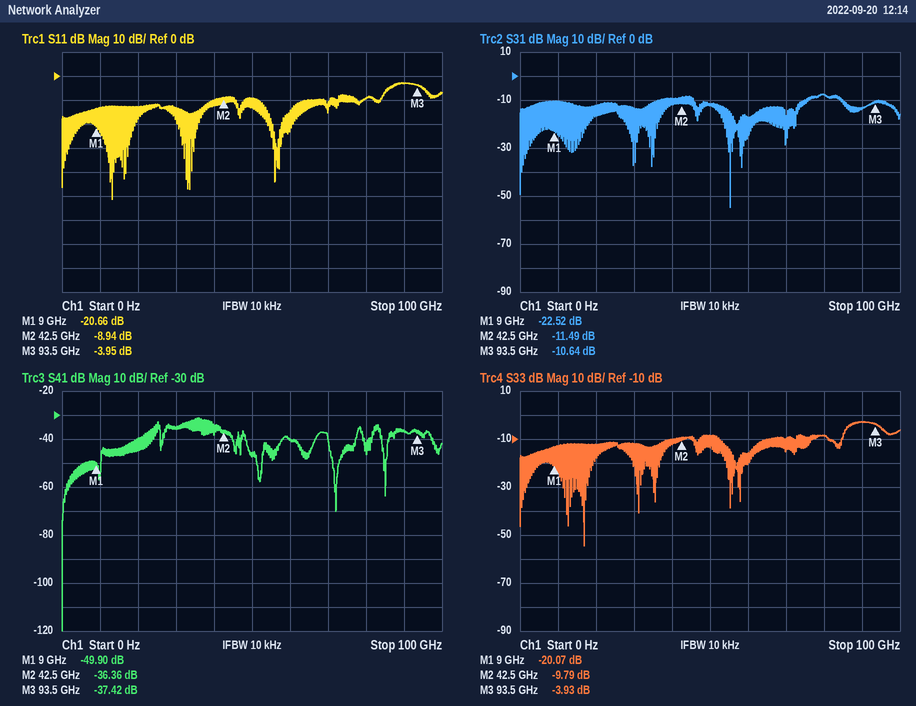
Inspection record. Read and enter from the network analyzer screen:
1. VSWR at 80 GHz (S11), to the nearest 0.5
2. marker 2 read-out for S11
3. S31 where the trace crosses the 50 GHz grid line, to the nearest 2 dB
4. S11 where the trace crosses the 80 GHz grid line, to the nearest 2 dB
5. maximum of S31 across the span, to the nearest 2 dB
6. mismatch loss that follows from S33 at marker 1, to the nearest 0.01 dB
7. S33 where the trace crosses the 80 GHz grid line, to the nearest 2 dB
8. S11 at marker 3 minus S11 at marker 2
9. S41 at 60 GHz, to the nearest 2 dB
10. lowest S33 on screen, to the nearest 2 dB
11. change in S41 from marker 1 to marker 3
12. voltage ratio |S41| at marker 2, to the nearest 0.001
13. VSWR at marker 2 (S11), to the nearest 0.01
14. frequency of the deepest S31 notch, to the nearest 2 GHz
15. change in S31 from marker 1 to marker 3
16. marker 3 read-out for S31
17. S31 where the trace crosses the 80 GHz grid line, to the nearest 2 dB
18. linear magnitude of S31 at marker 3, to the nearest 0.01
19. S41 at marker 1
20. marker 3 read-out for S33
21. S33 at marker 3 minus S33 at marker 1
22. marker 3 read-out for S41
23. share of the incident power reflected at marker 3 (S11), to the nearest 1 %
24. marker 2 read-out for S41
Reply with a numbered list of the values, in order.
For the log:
1. 2.0
2. -8.94 dB
3. -12 dB
4. -10 dB
5. -8 dB
6. 0.04 dB
7. -8 dB
8. 4.99 dB
9. -40 dB
10. -54 dB
11. 12.48 dB
12. 0.015
13. 2.11
14. 56 GHz
15. 11.88 dB
16. -10.64 dB
17. -8 dB
18. 0.29
19. -49.90 dB
20. -3.93 dB
21. 16.14 dB
22. -37.42 dB
23. 40 %
24. -36.36 dB
